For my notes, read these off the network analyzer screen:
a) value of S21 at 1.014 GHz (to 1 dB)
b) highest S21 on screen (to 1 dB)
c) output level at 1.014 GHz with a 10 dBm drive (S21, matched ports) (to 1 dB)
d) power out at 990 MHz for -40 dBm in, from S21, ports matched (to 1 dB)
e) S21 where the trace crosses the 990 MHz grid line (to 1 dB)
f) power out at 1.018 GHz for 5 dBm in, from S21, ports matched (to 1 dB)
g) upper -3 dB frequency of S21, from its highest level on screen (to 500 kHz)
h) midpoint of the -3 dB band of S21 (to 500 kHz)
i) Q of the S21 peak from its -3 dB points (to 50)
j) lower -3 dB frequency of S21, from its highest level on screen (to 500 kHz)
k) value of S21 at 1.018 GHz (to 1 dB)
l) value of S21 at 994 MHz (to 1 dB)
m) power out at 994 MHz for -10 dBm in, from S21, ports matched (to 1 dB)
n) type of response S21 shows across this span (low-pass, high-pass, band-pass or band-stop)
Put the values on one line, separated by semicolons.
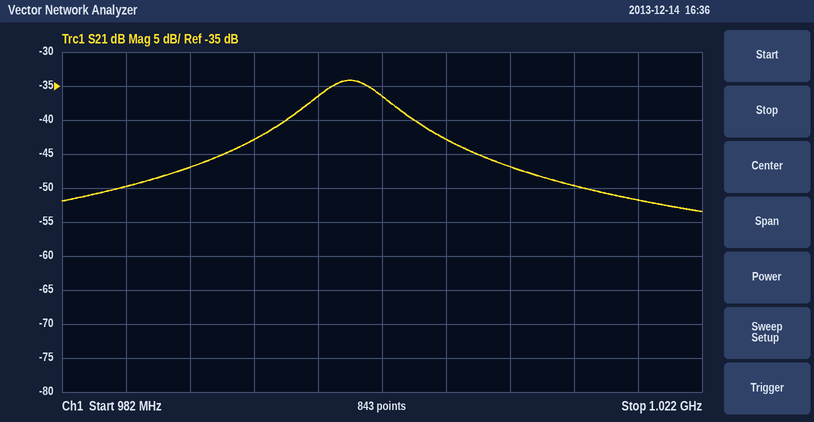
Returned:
-50 dB; -34 dB; -40 dBm; -87 dBm; -47 dB; -47 dBm; 1.0025 GHz; 1.0000 GHz; 200; 997.5 MHz; -52 dB; -43 dB; -53 dBm; band-pass
